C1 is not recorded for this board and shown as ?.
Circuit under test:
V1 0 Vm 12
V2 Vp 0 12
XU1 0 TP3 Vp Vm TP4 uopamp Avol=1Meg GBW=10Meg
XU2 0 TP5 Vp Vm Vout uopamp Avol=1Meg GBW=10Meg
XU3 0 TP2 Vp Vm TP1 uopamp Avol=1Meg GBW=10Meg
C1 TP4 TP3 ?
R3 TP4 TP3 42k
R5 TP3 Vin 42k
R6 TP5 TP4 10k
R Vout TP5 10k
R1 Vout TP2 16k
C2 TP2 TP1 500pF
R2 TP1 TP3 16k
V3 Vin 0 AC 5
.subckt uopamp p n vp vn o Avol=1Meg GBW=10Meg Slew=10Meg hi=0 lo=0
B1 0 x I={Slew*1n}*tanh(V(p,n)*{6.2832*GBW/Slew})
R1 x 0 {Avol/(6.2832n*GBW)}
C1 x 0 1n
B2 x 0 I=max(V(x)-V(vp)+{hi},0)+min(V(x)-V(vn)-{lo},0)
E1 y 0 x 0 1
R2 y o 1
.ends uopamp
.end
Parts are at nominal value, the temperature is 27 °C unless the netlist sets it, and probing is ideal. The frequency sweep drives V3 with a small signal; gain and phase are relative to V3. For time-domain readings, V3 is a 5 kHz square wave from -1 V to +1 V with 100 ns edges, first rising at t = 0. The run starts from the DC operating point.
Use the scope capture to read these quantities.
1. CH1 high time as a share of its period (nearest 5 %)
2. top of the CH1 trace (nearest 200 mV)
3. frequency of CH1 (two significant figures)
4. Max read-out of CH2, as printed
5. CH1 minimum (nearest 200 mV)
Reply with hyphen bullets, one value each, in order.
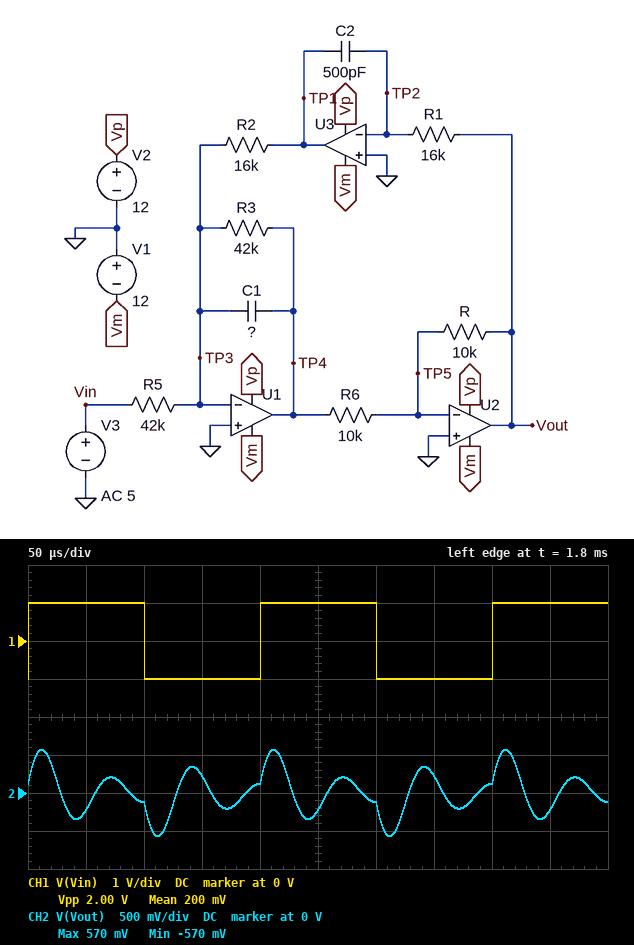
- 50 %
- 1.0 V
- 5.0 kHz
- 570 mV
- -1.0 V
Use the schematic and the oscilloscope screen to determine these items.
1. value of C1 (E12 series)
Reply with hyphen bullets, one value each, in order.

- 680 pF
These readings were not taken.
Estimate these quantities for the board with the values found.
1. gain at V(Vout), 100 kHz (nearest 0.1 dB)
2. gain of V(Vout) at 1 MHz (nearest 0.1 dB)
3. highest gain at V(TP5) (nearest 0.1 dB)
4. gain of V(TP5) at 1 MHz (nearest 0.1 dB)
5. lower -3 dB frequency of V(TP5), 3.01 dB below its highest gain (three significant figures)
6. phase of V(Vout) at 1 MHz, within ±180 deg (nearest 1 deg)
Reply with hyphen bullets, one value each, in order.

- -24.9 dB
- -45.3 dB
- -55.1 dB
- -65.3 dB
- 15.1 kHz
- -107 deg
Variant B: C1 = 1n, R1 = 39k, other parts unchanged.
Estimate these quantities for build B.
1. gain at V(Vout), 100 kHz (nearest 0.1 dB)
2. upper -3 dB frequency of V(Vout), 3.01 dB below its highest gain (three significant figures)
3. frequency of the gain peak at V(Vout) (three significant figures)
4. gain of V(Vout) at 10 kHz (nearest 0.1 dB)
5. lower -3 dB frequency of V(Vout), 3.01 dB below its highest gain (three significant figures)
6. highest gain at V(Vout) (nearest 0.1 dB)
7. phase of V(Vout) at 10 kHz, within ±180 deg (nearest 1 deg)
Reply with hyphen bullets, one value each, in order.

- -28.4 dB
- 11.1 kHz
- 9.00 kHz
- -0.9 dB
- 7.32 kHz
- 0.1 dB
- -27 deg
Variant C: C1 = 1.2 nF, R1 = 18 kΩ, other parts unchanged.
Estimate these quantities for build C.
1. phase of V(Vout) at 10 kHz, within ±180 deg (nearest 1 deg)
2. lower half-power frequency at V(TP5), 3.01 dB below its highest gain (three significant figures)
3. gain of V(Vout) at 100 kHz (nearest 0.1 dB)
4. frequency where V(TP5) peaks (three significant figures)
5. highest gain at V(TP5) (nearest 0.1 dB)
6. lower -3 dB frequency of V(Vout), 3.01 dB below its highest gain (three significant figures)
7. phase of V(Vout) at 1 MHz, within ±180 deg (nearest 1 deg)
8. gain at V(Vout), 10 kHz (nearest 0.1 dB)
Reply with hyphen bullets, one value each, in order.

- 56 deg
- 10.9 kHz
- -29.9 dB
- 12.3 kHz
- -58.1 dB
- 10.6 kHz
- -107 deg
- -4.9 dB
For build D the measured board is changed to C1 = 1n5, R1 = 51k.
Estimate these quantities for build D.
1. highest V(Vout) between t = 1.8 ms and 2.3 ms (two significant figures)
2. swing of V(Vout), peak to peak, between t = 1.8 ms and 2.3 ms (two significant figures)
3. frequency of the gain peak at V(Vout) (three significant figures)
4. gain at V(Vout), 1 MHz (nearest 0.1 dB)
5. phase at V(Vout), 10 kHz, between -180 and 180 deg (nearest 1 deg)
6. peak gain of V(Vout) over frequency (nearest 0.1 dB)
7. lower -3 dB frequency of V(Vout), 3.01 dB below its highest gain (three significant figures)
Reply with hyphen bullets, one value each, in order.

- 850 mV
- 1.7 V
- 6.43 kHz
- -52.2 dB
- -67 deg
- 0.1 dB
- 5.30 kHz
